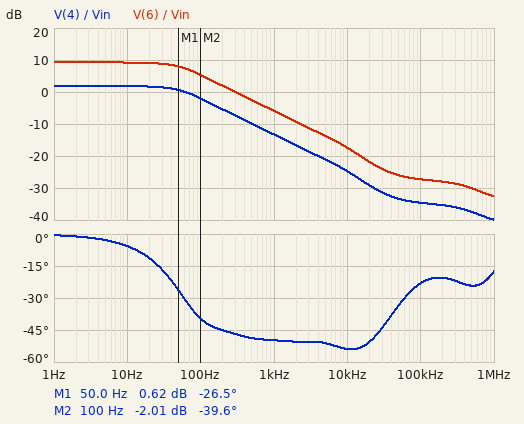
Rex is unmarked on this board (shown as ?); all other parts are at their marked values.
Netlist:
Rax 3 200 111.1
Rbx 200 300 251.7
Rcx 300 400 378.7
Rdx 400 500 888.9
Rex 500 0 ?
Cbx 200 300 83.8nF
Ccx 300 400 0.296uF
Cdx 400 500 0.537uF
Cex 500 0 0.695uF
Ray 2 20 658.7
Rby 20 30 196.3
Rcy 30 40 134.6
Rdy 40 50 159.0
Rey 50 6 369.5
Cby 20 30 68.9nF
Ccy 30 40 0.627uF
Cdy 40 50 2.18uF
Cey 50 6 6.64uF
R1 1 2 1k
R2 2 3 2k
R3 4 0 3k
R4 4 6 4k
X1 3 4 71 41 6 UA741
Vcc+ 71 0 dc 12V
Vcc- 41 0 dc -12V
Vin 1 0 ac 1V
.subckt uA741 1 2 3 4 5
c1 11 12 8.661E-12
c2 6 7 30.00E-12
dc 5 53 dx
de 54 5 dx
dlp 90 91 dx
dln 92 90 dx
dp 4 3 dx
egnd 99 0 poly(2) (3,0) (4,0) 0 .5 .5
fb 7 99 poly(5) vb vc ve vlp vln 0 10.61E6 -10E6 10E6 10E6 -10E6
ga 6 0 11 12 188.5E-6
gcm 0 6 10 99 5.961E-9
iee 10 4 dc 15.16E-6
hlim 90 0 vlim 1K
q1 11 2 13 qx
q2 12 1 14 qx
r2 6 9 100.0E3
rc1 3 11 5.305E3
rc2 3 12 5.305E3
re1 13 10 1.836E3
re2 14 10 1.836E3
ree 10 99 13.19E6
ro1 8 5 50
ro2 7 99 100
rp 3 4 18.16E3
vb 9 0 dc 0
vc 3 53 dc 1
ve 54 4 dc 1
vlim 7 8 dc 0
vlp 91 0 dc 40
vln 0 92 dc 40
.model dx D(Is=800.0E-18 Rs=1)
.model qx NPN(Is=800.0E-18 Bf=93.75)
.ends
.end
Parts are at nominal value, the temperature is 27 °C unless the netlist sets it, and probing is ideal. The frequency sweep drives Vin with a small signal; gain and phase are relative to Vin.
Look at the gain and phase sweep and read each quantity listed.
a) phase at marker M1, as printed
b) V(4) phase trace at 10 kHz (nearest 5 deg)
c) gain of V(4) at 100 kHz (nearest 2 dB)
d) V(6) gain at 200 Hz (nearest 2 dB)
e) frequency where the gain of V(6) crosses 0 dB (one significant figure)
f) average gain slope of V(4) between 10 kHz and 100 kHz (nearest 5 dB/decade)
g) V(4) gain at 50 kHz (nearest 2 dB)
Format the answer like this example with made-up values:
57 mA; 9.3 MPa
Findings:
-26.5 deg; -55 deg; -34 dB; 2 dB; 300 Hz; -10 dB/decade; -34 dB
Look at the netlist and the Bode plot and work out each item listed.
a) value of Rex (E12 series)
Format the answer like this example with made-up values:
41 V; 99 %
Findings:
4.7 kΩ
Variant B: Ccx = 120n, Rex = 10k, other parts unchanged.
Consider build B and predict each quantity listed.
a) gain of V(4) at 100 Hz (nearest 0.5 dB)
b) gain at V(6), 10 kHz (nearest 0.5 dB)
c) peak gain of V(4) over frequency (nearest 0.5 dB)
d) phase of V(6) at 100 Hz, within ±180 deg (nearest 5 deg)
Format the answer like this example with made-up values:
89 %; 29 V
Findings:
-2.0 dB; -15.5 dB; 6.0 dB; -50 deg
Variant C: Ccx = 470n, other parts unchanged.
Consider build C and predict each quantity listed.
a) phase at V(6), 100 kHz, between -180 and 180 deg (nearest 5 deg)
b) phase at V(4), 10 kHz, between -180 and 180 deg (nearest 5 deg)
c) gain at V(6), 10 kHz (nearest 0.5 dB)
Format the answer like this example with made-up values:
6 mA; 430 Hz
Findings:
-20 deg; -50 deg; -18.0 dB
